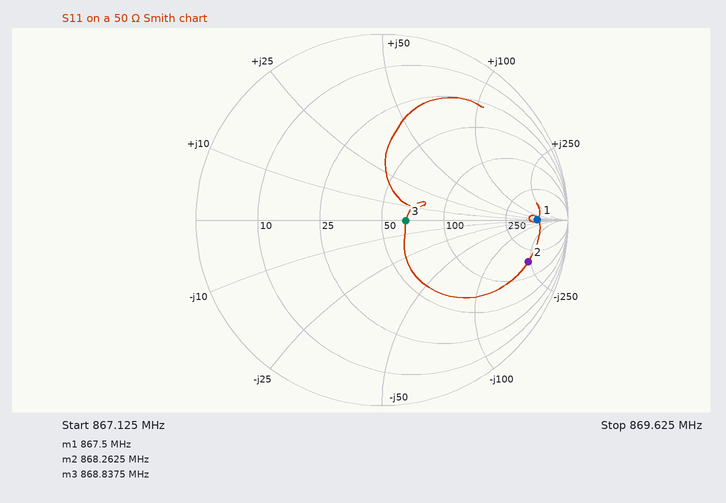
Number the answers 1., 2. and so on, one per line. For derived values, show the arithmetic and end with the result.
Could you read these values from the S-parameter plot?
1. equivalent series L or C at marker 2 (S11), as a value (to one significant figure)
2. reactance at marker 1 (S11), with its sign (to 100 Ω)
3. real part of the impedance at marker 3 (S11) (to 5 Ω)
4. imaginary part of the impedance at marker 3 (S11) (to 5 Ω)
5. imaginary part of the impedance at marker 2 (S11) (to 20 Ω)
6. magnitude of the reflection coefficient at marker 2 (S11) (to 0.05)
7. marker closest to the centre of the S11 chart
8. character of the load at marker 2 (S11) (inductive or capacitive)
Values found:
1. C = 1/(2π × 868.2625 MHz × 240 Ω) ≈ 764 fF, so 800 fF to one significant figure
2. 0 Ω
3. 65 Ω
4. 0 Ω
5. -240 Ω
6. 0.80
7. marker 3
8. capacitive
